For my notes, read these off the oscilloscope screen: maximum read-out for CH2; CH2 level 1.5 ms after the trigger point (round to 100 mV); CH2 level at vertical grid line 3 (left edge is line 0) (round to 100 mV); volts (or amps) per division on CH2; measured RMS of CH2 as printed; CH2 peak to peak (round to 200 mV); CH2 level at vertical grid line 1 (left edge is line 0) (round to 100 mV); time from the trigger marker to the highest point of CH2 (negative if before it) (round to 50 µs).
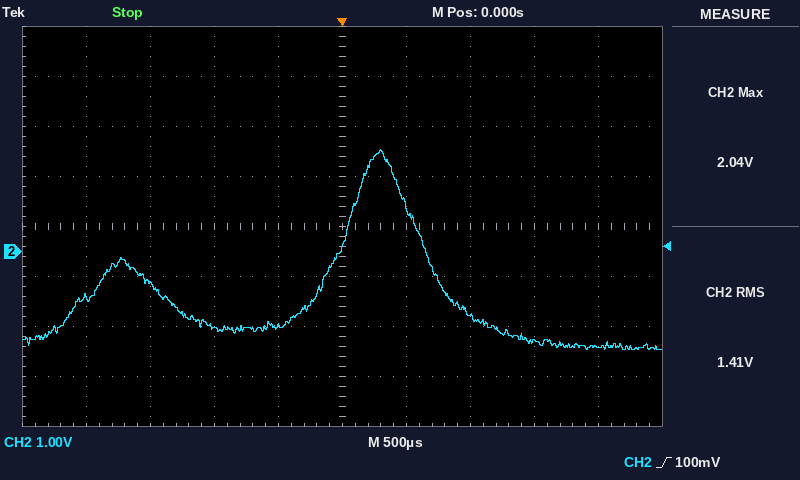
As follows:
2.04 V
-1.8 V
-1.5 V
1 V
1.41 V
4.0 V
-900 mV
+300 µs
